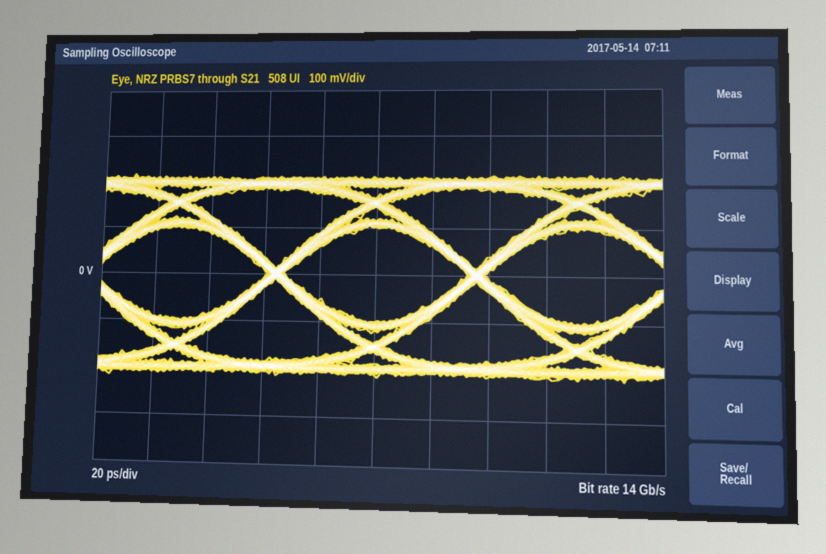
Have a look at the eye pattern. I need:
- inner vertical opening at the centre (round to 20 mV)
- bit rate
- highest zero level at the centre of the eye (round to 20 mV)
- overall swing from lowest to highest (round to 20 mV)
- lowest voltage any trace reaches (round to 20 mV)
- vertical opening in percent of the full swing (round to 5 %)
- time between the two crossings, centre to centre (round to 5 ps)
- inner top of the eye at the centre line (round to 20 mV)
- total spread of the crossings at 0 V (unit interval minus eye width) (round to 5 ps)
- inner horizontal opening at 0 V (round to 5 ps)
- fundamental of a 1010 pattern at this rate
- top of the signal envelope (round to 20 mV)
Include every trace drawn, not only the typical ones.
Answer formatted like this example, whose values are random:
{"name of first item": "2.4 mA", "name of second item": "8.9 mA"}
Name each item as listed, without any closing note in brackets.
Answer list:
{"inner vertical opening at the centre": "200 mV", "bit rate": "14 Gb/s", "highest zero level at the centre of the eye": "-100 mV", "overall swing from lowest to highest": "440 mV", "lowest voltage any trace reaches": "-220 mV", "vertical opening in percent of the full swing": "45 %", "time between the two crossings, centre to centre": "70 ps", "inner top of the eye at the centre line": "100 mV", "total spread of the crossings at 0 V (unit interval minus eye width)": "5 ps", "inner horizontal opening at 0 V": "65 ps", "fundamental of a 1010 pattern at this rate": "7 GHz", "top of the signal envelope": "220 mV"}
